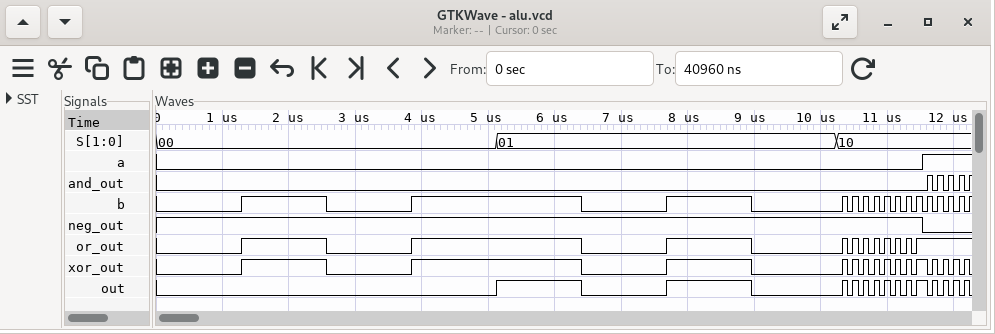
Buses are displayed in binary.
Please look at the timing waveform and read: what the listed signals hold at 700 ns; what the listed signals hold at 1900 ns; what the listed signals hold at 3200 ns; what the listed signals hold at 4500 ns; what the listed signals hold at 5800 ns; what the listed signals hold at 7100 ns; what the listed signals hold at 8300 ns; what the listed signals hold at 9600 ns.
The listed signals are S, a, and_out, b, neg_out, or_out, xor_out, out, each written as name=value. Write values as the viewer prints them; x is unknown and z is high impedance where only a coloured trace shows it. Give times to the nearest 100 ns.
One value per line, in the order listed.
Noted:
S=00, a=0, and_out=0, b=0, neg_out=1, or_out=0, xor_out=0, out=0
S=00, a=0, and_out=0, b=1, neg_out=1, or_out=1, xor_out=1, out=0
S=00, a=0, and_out=0, b=0, neg_out=1, or_out=0, xor_out=0, out=0
S=00, a=0, and_out=0, b=1, neg_out=1, or_out=1, xor_out=1, out=0
S=01, a=0, and_out=0, b=1, neg_out=1, or_out=1, xor_out=1, out=1
S=01, a=0, and_out=0, b=0, neg_out=1, or_out=0, xor_out=0, out=0
S=01, a=0, and_out=0, b=1, neg_out=1, or_out=1, xor_out=1, out=1
S=01, a=0, and_out=0, b=0, neg_out=1, or_out=0, xor_out=0, out=0
